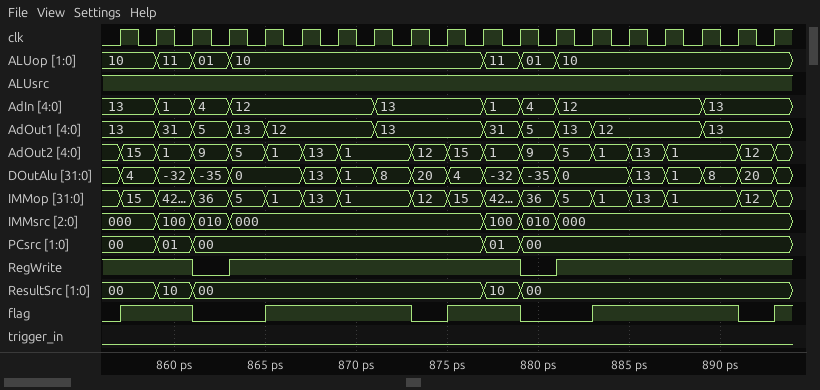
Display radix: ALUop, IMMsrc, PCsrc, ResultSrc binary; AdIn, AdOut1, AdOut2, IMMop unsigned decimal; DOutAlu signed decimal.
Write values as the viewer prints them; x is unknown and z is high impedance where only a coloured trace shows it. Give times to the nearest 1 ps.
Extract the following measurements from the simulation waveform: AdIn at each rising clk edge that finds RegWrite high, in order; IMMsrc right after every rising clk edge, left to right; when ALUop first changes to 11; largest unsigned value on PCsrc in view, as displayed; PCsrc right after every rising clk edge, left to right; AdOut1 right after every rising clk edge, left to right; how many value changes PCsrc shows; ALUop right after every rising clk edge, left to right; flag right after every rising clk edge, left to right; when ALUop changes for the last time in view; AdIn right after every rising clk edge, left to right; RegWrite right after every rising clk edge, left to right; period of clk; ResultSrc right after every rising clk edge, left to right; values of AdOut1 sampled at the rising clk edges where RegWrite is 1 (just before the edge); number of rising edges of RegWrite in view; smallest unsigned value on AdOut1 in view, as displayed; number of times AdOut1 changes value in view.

13, 13, 1, 12, 12, 12, 12, 13, 13, 13, 1, 12, 12, 12, 12, 13, 13
000, 100, 010, 000, 000, 000, 000, 000, 000, 000, 100, 010, 000, 000, 000, 000, 000, 000, 000
859 ps
01
00, 01, 00, 00, 00, 00, 00, 00, 00, 00, 01, 00, 00, 00, 00, 00, 00, 00, 00
13, 31, 5, 13, 12, 12, 12, 13, 13, 13, 31, 5, 13, 12, 12, 12, 13, 13, 13
4
10, 11, 01, 10, 10, 10, 10, 10, 10, 10, 11, 01, 10, 10, 10, 10, 10, 10, 10
1 1 0 0 1 1 1 1 0 1 1 0 0 1 1 1 1 0 1
881 ps
13, 1, 4, 12, 12, 12, 12, 13, 13, 13, 1, 4, 12, 12, 12, 12, 13, 13, 13
1 1 0 1 1 1 1 1 1 1 1 0 1 1 1 1 1 1 1
2 ps
00, 10, 00, 00, 00, 00, 00, 00, 00, 00, 10, 00, 00, 00, 00, 00, 00, 00, 00
13, 13, 31, 13, 12, 12, 12, 13, 13, 13, 31, 13, 12, 12, 12, 13, 13
2
5
10
